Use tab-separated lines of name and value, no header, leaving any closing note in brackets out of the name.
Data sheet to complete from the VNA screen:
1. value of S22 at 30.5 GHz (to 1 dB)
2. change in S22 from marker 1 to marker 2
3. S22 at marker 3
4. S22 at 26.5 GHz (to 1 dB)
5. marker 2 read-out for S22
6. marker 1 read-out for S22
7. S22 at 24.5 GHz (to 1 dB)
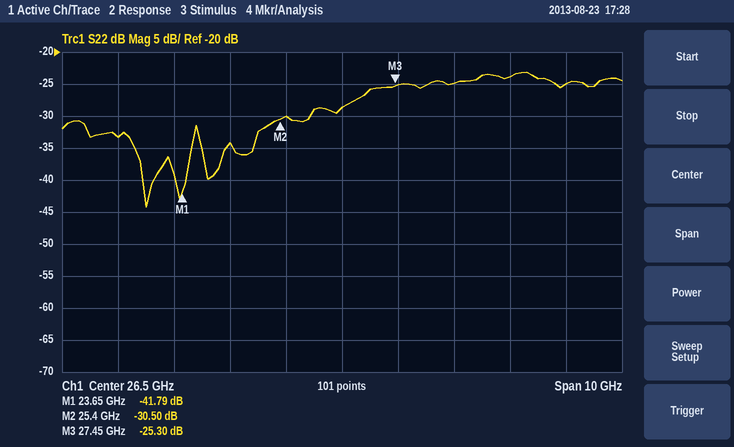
value of S22 at 30.5 GHz	-25 dB
change in S22 from marker 1 to marker 2	11.29 dB
S22 at marker 3	-25.30 dB
S22 at 26.5 GHz	-29 dB
marker 2 read-out for S22	-30.50 dB
marker 1 read-out for S22	-41.79 dB
S22 at 24.5 GHz	-34 dB
